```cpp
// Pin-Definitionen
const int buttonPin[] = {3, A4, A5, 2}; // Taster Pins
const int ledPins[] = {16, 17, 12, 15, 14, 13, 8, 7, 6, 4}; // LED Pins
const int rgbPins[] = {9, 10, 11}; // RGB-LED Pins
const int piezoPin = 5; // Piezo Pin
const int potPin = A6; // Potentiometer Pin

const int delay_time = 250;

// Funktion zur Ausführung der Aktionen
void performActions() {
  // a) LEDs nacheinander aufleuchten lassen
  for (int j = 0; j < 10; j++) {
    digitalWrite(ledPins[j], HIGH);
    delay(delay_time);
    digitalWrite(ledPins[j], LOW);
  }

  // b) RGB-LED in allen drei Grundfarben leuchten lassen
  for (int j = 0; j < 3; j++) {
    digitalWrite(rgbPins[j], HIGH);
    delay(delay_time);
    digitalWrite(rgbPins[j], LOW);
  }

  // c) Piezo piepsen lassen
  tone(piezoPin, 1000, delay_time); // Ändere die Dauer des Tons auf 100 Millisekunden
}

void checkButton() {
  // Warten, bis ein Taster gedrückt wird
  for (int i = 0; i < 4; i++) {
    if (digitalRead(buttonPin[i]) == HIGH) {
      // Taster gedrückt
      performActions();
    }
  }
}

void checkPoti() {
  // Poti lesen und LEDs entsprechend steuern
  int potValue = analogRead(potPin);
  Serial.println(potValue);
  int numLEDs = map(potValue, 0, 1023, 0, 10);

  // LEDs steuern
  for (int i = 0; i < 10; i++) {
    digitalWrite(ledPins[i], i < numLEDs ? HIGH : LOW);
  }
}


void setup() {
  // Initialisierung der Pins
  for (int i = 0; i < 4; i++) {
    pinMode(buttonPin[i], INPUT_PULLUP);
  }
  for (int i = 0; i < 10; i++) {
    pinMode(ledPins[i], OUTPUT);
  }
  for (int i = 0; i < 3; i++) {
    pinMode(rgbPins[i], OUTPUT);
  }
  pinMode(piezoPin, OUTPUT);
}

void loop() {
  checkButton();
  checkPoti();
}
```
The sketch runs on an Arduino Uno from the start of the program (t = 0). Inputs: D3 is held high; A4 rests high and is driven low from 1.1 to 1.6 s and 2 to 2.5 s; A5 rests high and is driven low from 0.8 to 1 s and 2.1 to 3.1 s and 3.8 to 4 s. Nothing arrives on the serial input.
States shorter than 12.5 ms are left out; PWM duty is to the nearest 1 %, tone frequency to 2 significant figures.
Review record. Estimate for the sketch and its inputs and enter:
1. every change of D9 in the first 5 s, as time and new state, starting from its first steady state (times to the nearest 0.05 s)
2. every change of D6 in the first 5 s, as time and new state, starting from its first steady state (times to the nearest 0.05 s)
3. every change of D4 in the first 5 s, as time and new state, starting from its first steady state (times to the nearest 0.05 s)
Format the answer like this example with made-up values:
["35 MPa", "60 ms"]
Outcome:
["0 s low; 2.5 s high; 2.75 s low", "0 s low; 2 s high; 2.25 s low", "0 s low; 2.25 s high; 2.5 s low"]
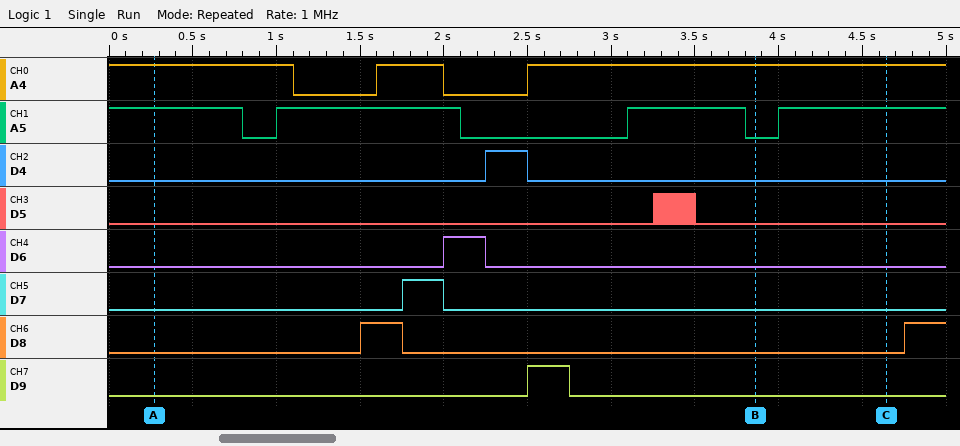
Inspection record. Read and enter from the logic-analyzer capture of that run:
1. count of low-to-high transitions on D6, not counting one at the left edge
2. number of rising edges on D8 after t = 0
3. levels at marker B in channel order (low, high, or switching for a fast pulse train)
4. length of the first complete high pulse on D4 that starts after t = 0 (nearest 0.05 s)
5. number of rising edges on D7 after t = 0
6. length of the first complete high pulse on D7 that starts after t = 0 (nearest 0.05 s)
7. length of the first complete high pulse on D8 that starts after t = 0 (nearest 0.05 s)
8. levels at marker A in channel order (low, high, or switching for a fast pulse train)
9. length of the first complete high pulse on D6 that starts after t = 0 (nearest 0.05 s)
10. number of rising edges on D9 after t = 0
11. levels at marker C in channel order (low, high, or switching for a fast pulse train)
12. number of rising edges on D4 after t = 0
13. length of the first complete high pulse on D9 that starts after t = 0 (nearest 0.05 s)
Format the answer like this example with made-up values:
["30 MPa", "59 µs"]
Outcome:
["1", "2", "A4 high, A5 low, D4 low, D5 low, D6 low, D7 low, D8 low, D9 low", "0.25 s", "1", "0.25 s", "0.25 s", "A4 high, A5 high, D4 low, D5 low, D6 low, D7 low, D8 low, D9 low", "0.25 s", "1", "A4 high, A5 high, D4 low, D5 low, D6 low, D7 low, D8 low, D9 low", "1", "0.25 s"]
